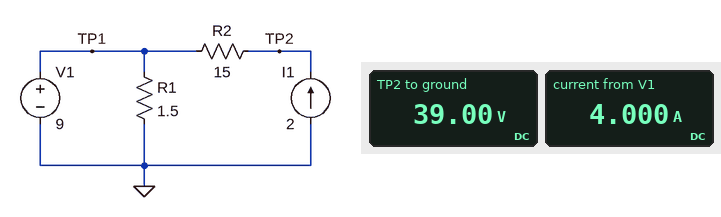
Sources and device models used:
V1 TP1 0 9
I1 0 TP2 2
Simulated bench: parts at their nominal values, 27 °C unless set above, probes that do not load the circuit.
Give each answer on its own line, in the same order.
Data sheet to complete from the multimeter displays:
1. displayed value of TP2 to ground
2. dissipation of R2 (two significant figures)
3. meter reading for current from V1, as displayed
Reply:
39.00 V
60 W
4.000 A
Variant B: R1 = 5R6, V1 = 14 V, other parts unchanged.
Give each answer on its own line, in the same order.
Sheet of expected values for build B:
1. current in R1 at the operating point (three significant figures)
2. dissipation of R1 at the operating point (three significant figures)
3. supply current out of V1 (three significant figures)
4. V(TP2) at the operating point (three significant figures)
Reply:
2.50 A
35.0 W
500 mA
44.0 V
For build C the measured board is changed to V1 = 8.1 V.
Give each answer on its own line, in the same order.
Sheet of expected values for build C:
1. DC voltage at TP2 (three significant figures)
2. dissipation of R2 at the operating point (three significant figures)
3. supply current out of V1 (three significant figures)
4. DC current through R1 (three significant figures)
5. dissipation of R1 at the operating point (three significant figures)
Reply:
38.1 V
60.0 W
3.40 A
5.40 A
43.7 W
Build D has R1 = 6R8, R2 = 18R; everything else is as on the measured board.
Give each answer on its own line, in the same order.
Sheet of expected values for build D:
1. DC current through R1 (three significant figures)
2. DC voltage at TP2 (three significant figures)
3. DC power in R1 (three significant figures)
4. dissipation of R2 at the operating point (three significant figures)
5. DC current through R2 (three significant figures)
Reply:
1.32 A
45.0 V
11.9 W
72.0 W
2.00 A
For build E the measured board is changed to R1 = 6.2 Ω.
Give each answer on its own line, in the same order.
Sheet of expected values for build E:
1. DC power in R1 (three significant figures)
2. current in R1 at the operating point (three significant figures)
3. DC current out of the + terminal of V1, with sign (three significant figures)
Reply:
13.1 W
1.45 A
-548 mA
